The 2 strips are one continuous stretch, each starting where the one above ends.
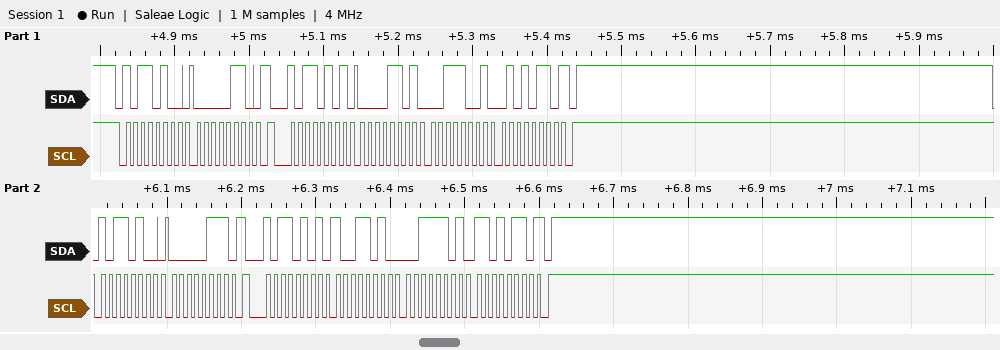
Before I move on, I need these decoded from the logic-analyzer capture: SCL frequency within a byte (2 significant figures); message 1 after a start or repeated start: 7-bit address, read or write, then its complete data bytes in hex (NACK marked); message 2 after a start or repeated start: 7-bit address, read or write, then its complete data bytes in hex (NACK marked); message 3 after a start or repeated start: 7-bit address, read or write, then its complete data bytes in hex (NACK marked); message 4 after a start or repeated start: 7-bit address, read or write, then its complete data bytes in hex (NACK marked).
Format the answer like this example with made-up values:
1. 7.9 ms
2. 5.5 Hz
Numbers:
1. 100 kHz
2. 0x5A write: 06
3. 0x5A read: 0D 39 56 NACK
4. 0x5A write: 07
5. 0x5A read: 9A 3D D6 NACK
